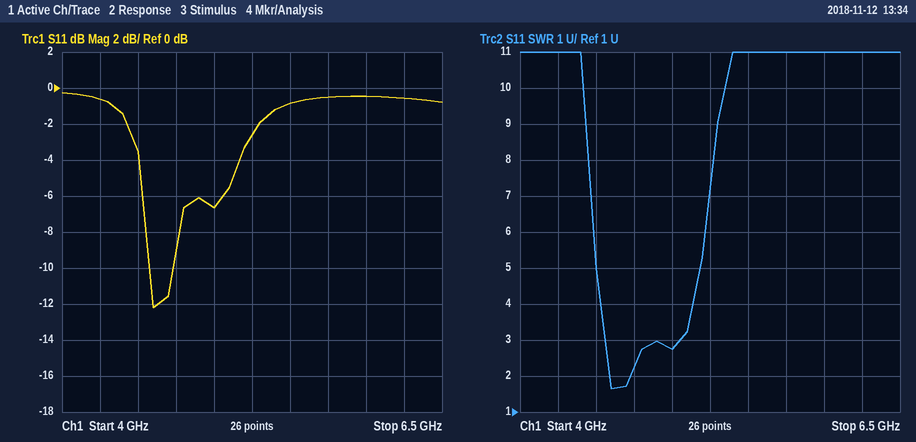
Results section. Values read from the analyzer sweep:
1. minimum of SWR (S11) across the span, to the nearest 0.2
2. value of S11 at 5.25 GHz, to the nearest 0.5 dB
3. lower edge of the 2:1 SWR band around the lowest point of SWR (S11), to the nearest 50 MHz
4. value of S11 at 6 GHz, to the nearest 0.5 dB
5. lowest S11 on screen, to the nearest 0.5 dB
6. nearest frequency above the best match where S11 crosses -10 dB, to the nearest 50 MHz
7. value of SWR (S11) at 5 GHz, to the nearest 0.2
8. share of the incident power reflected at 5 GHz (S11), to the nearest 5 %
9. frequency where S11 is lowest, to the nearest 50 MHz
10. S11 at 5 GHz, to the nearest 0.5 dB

1.6
-2.5 dB
4.60 GHz
-0.5 dB
-12.0 dB
4.75 GHz
2.8
20 %
4.60 GHz
-6.5 dB
